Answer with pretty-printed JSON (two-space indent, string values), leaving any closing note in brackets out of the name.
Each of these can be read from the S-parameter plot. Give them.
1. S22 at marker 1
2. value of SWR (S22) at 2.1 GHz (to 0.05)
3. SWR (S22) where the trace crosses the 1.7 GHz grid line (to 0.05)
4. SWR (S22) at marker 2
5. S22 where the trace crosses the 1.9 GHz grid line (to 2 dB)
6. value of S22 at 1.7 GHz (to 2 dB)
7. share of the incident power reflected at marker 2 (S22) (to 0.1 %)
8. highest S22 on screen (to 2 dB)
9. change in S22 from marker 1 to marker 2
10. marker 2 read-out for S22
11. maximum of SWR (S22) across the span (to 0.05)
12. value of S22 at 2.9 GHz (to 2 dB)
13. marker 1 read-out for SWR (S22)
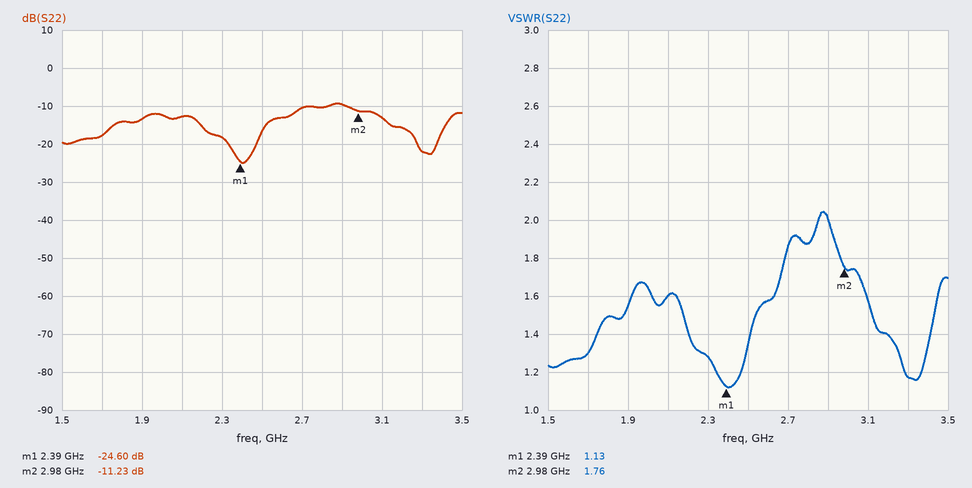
{
  "S22 at marker 1": "-24.60 dB",
  "value of SWR (S22) at 2.1 GHz": "1.60",
  "SWR (S22) where the trace crosses the 1.7 GHz grid line": "1.30",
  "SWR (S22) at marker 2": "1.76",
  "S22 where the trace crosses the 1.9 GHz grid line": "-14 dB",
  "value of S22 at 1.7 GHz": "-18 dB",
  "share of the incident power reflected at marker 2 (S22)": "7.5 %",
  "highest S22 on screen": "-10 dB",
  "change in S22 from marker 1 to marker 2": "13.37 dB",
  "marker 2 read-out for S22": "-11.23 dB",
  "maximum of SWR (S22) across the span": "2.05",
  "value of S22 at 2.9 GHz": "-10 dB",
  "marker 1 read-out for SWR": "1.13"
}
